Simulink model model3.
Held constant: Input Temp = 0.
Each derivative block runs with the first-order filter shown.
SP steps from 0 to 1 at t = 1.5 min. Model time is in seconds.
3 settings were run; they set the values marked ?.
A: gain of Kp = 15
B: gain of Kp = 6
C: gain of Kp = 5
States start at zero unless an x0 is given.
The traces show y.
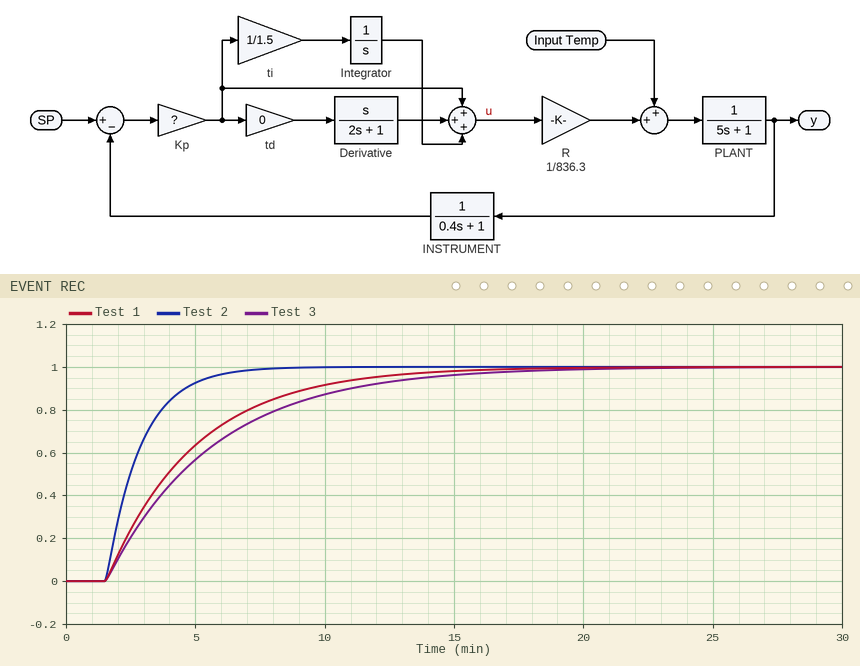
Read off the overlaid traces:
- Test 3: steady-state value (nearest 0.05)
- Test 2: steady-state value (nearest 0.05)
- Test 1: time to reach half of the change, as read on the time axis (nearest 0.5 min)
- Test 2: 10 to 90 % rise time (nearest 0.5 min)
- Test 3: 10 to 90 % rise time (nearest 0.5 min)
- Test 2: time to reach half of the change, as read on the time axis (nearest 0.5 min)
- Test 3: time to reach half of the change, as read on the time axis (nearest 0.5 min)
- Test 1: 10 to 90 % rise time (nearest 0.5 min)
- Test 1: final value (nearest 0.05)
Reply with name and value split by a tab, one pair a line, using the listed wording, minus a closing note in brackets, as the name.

Test 3: steady-state value	1.00
Test 2: steady-state value	1.00
Test 1: time to reach half of the change, as read on the time axis	4.0 min
Test 2: 10 to 90 % rise time	3.0 min
Test 3: 10 to 90 % rise time	9.0 min
Test 2: time to reach half of the change, as read on the time axis	2.5 min
Test 3: time to reach half of the change, as read on the time axis	4.5 min
Test 1: 10 to 90 % rise time	7.5 min
Test 1: final value	1.00
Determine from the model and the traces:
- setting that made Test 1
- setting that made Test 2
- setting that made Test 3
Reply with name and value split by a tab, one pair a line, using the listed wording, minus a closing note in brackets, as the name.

setting that made Test 1	B
setting that made Test 2	A
setting that made Test 3	C
